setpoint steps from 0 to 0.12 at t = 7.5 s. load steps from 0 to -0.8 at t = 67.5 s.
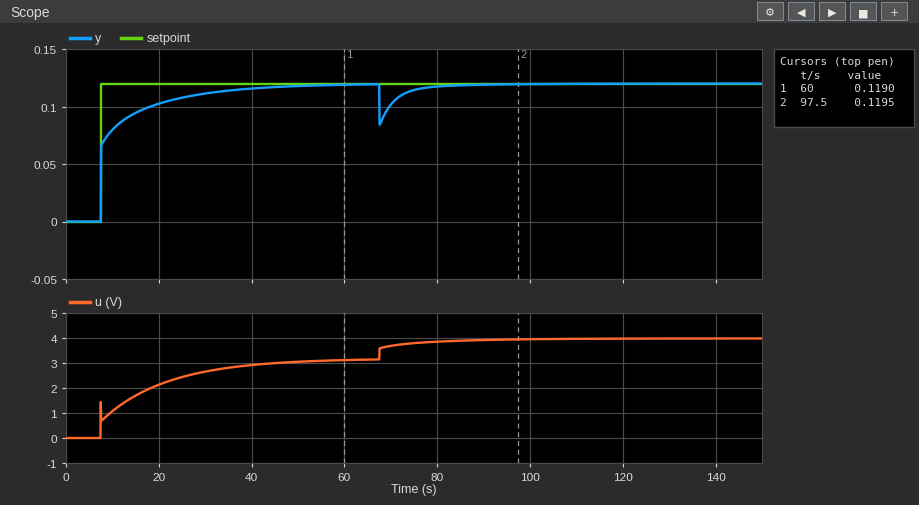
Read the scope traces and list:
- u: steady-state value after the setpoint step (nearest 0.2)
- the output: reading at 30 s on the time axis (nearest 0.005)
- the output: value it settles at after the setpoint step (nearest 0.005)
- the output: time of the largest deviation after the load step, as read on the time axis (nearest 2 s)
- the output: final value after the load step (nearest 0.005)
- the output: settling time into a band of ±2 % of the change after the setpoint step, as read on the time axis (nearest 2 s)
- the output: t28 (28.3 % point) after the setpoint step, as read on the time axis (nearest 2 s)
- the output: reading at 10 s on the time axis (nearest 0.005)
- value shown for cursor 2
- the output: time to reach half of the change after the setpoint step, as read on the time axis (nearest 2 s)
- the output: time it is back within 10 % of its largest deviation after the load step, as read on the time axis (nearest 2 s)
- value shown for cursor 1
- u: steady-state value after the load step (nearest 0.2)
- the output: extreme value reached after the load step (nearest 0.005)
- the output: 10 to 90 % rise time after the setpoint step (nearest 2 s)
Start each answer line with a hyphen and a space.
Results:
- 3.2
- 0.110
- 0.120
- 68 s
- 0.120
- 48 s
- 8 s
- 0.080
- 0.1195
- 8 s
- 78 s
- 0.1190
- 4.0
- 0.085
- 18 s
